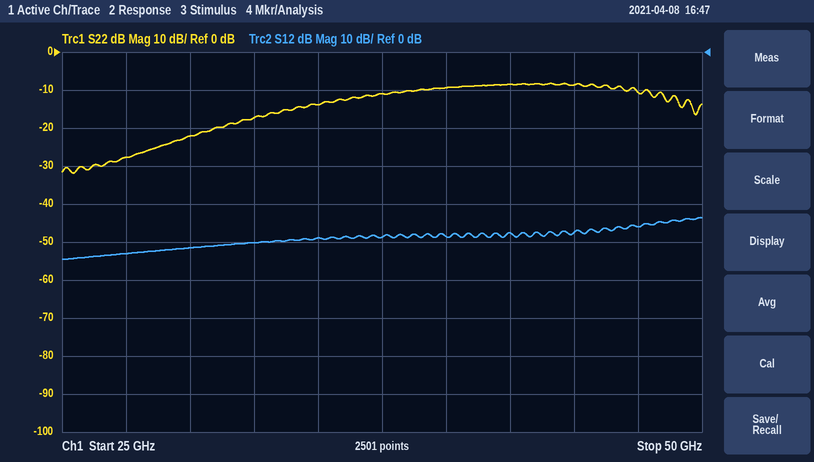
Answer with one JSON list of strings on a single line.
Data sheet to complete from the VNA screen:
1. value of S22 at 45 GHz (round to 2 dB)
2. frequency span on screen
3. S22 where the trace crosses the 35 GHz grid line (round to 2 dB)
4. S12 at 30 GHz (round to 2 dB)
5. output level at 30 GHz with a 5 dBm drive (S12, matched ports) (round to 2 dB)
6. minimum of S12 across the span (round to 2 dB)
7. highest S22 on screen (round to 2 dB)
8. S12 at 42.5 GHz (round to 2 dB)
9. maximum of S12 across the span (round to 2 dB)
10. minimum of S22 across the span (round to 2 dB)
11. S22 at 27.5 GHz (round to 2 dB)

["-8 dB", "25 GHz", "-14 dB", "-52 dB", "-46 dBm", "-54 dB", "-8 dB", "-48 dB", "-44 dB", "-32 dB", "-28 dB"]
